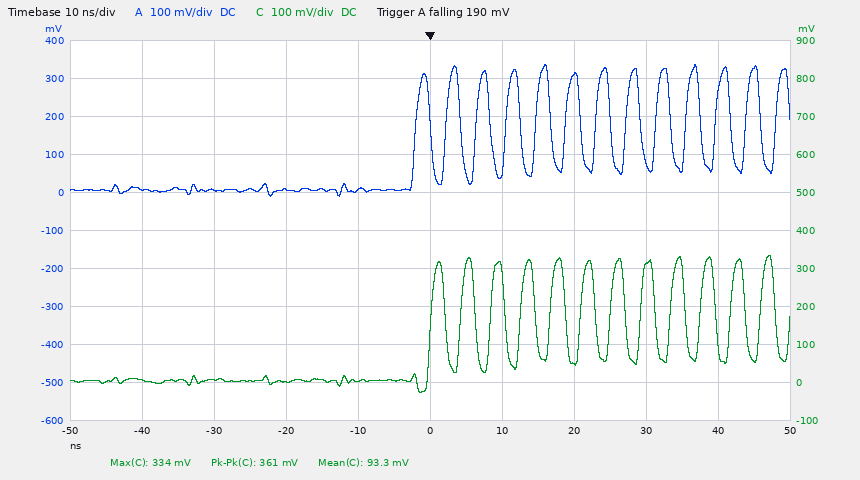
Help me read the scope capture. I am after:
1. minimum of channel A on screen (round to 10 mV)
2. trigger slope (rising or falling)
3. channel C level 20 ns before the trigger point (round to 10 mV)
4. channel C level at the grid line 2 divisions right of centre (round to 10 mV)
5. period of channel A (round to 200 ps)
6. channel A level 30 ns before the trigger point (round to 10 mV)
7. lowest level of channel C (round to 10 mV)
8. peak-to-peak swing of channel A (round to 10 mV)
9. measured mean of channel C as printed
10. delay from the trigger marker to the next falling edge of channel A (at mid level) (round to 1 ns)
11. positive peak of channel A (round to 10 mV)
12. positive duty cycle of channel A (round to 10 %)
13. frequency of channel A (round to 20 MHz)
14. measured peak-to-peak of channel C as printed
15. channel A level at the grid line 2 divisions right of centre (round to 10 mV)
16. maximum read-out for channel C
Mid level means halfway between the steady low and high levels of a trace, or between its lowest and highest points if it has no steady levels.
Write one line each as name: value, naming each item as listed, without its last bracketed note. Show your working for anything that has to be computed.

minimum of channel A on screen: -10 mV
trigger slope: falling
channel C level 20 ns before the trigger point: 0 mV
channel C level at the grid line 2 divisions right of centre: 50 mV
period of channel A: 4.2 ns
channel A level 30 ns before the trigger point: 10 mV
lowest level of channel C: -30 mV
peak-to-peak swing of channel A: 340 mV − (-10 mV) = 350 mV
measured mean of channel C as printed: 93.3 mV
delay from the trigger marker to the next falling edge of channel A (at mid level): 4 ns
positive peak of channel A: 340 mV
positive duty cycle of channel A: 50 %
frequency of channel A: 1 / 4.2 ns ≈ 238 MHz, so 240 MHz to the nearest 20 MHz
measured peak-to-peak of channel C as printed: 361 mV
channel A level at the grid line 2 divisions right of centre: 310 mV
maximum read-out for channel C: 334 mV
